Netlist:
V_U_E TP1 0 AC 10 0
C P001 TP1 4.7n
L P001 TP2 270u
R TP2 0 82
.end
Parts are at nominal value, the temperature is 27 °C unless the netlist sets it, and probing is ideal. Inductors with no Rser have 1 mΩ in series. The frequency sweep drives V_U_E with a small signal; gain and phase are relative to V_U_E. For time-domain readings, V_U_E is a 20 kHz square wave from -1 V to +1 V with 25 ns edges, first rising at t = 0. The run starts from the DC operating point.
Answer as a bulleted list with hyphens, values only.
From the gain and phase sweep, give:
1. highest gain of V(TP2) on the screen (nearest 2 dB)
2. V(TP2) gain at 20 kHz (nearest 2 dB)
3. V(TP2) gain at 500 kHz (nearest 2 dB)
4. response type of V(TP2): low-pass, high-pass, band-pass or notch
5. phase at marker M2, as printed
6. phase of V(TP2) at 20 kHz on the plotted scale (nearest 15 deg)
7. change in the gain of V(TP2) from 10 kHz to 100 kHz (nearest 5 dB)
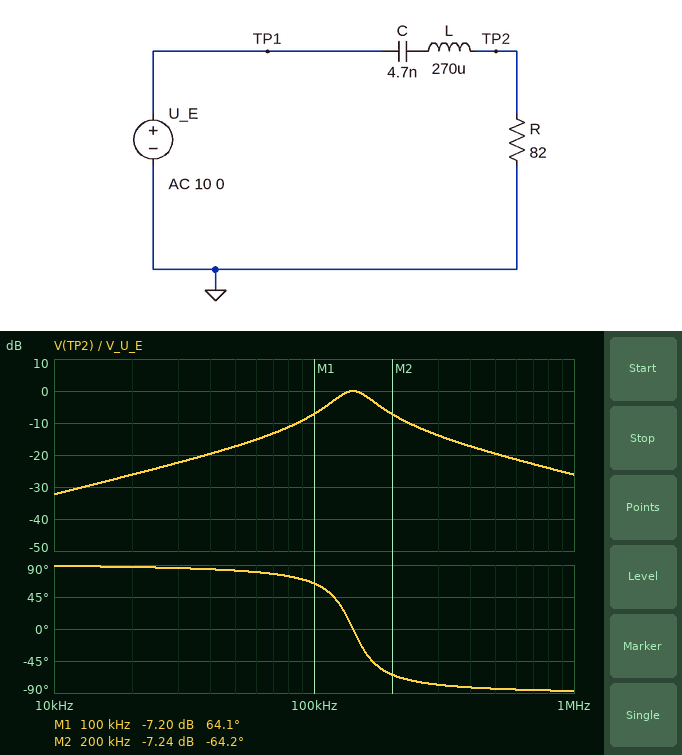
- 0 dB
- -26 dB
- -20 dB
- band-pass
- -64.2 deg
- 90 deg
- 25 dB
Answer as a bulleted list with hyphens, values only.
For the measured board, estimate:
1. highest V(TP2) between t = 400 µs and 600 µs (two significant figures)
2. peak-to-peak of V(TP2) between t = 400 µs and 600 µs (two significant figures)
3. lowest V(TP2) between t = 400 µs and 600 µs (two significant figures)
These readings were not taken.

- 550 mV
- 1.1 V
- -550 mV
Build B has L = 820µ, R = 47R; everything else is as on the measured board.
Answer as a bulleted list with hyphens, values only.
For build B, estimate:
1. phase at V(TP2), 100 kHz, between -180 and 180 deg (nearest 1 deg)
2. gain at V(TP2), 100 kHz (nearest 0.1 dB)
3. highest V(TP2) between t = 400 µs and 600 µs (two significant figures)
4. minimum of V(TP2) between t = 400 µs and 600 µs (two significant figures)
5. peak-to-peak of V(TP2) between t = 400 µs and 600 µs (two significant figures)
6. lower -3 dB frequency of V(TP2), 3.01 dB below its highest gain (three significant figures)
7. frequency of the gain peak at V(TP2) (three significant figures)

- -75 deg
- -11.8 dB
- 140 mV
- -140 mV
- 280 mV
- 76.6 kHz
- 81.1 kHz
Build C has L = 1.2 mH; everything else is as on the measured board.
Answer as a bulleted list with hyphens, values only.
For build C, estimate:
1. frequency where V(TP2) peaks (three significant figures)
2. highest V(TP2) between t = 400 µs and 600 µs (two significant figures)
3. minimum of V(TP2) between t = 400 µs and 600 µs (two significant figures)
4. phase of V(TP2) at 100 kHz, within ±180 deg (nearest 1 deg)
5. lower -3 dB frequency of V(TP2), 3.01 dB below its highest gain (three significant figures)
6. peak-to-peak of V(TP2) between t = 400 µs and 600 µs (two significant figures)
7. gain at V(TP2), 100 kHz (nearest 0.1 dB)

- 67.0 kHz
- 340 mV
- -340 mV
- -79 deg
- 61.8 kHz
- 680 mV
- -14.3 dB
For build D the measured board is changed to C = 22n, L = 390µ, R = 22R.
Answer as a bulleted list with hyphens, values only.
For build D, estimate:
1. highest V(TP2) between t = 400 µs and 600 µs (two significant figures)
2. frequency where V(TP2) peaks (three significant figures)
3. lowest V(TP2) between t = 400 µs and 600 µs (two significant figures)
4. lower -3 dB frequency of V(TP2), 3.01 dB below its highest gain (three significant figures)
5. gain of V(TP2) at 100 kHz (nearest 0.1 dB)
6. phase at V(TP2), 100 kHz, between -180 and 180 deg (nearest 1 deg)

- 350 mV
- 54.3 kHz
- -350 mV
- 50.0 kHz
- -18.0 dB
- -83 deg
